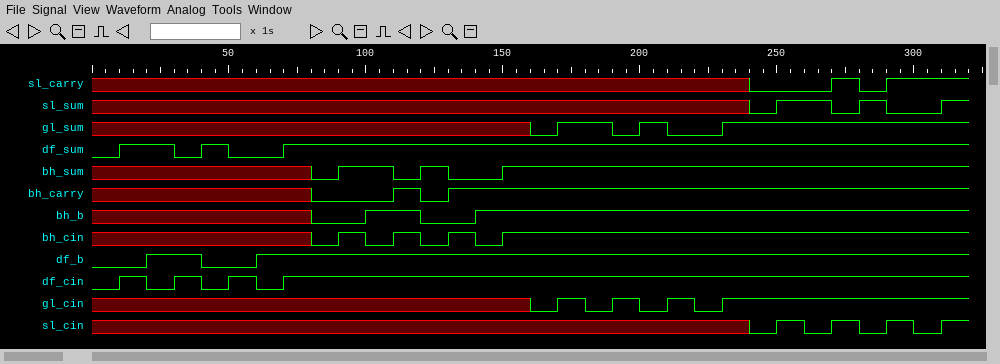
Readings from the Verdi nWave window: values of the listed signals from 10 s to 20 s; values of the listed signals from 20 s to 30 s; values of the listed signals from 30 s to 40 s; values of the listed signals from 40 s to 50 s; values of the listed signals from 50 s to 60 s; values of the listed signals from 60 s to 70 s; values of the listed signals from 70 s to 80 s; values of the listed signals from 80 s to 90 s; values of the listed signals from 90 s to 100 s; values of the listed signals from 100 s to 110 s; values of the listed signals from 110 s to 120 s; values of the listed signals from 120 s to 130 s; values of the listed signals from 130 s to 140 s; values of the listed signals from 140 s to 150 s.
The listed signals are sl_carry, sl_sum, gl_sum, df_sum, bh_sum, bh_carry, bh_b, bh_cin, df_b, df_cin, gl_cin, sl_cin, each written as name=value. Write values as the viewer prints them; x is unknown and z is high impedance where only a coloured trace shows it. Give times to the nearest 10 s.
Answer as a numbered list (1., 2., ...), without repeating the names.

1. sl_carry=x, sl_sum=x, gl_sum=x, df_sum=1, bh_sum=x, bh_carry=x, bh_b=x, bh_cin=x, df_b=0, df_cin=1, gl_cin=x, sl_cin=x
2. sl_carry=x, sl_sum=x, gl_sum=x, df_sum=1, bh_sum=x, bh_carry=x, bh_b=x, bh_cin=x, df_b=1, df_cin=0, gl_cin=x, sl_cin=x
3. sl_carry=x, sl_sum=x, gl_sum=x, df_sum=0, bh_sum=x, bh_carry=x, bh_b=x, bh_cin=x, df_b=1, df_cin=1, gl_cin=x, sl_cin=x
4. sl_carry=x, sl_sum=x, gl_sum=x, df_sum=1, bh_sum=x, bh_carry=x, bh_b=x, bh_cin=x, df_b=0, df_cin=0, gl_cin=x, sl_cin=x
5. sl_carry=x, sl_sum=x, gl_sum=x, df_sum=0, bh_sum=x, bh_carry=x, bh_b=x, bh_cin=x, df_b=0, df_cin=1, gl_cin=x, sl_cin=x
6. sl_carry=x, sl_sum=x, gl_sum=x, df_sum=0, bh_sum=x, bh_carry=x, bh_b=x, bh_cin=x, df_b=1, df_cin=0, gl_cin=x, sl_cin=x
7. sl_carry=x, sl_sum=x, gl_sum=x, df_sum=1, bh_sum=x, bh_carry=x, bh_b=x, bh_cin=x, df_b=1, df_cin=1, gl_cin=x, sl_cin=x
8. sl_carry=x, sl_sum=x, gl_sum=x, df_sum=1, bh_sum=0, bh_carry=0, bh_b=0, bh_cin=0, df_b=1, df_cin=1, gl_cin=x, sl_cin=x
9. sl_carry=x, sl_sum=x, gl_sum=x, df_sum=1, bh_sum=1, bh_carry=0, bh_b=0, bh_cin=1, df_b=1, df_cin=1, gl_cin=x, sl_cin=x
10. sl_carry=x, sl_sum=x, gl_sum=x, df_sum=1, bh_sum=1, bh_carry=0, bh_b=1, bh_cin=0, df_b=1, df_cin=1, gl_cin=x, sl_cin=x
11. sl_carry=x, sl_sum=x, gl_sum=x, df_sum=1, bh_sum=0, bh_carry=1, bh_b=1, bh_cin=1, df_b=1, df_cin=1, gl_cin=x, sl_cin=x
12. sl_carry=x, sl_sum=x, gl_sum=x, df_sum=1, bh_sum=1, bh_carry=0, bh_b=0, bh_cin=0, df_b=1, df_cin=1, gl_cin=x, sl_cin=x
13. sl_carry=x, sl_sum=x, gl_sum=x, df_sum=1, bh_sum=0, bh_carry=1, bh_b=0, bh_cin=1, df_b=1, df_cin=1, gl_cin=x, sl_cin=x
14. sl_carry=x, sl_sum=x, gl_sum=x, df_sum=1, bh_sum=0, bh_carry=1, bh_b=1, bh_cin=0, df_b=1, df_cin=1, gl_cin=x, sl_cin=x
